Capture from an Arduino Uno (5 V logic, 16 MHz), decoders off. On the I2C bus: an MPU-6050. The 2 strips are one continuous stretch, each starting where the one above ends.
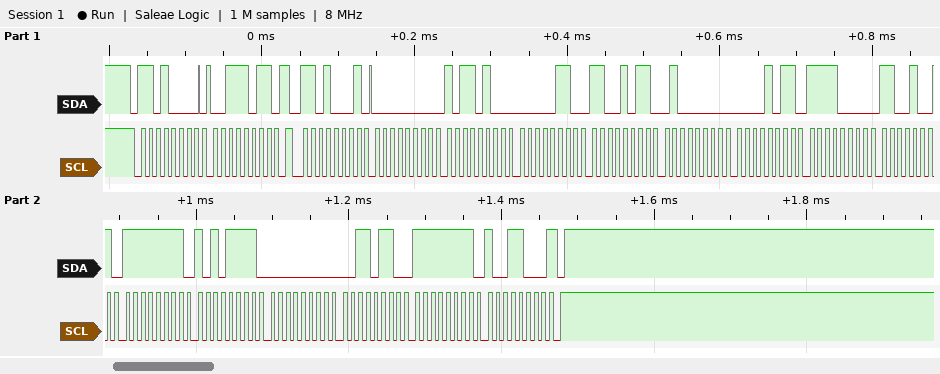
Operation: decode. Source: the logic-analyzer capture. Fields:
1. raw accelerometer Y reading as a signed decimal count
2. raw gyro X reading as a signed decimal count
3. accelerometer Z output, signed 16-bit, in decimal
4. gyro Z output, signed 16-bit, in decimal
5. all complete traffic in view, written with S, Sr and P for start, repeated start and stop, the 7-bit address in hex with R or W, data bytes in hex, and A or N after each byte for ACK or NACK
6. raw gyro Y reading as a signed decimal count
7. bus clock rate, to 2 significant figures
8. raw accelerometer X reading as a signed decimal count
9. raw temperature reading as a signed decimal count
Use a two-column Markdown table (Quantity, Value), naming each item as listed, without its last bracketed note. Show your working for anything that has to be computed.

| Quantity | Value |
|---|---|
| raw accelerometer Y reading as a signed decimal count | 0x06CB = 1739 |
| raw gyro X reading as a signed decimal count | 0xFFAF = -81 |
| accelerometer Z output, signed 16-bit, in decimal | 0x400B = 16395 |
| gyro Z output, signed 16-bit, in decimal | 0xFF98 = -104 |
| all complete traffic in view, written with S, Sr and P for start, repeated start and stop, the 7-bit address in hex with R or W, data bytes in hex, and A or N after each byte for ACK or NACK | S 68W A 3B A Sr 68R A 00 A B4 A 06 A CB A 40 A 0B A F0 A C9 A FF A AF A 00 A 36 A FF A 98 N P |
| raw gyro Y reading as a signed decimal count | 0x0036 = 54 |
| bus clock rate, to 2 significant figures | 100 kHz |
| raw accelerometer X reading as a signed decimal count | 0x00B4 = 180 |
| raw temperature reading as a signed decimal count | 0xF0C9 = -3895 |
